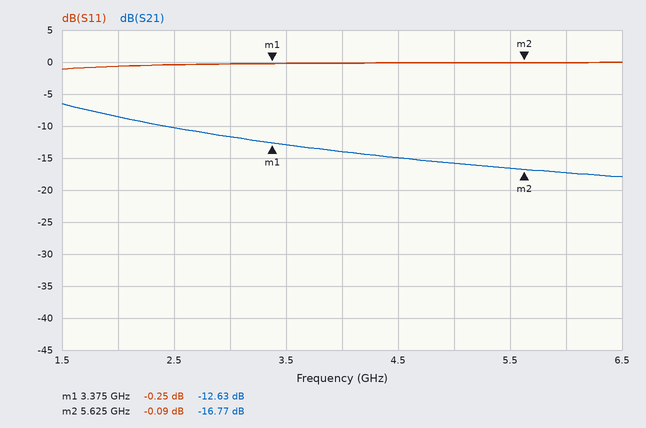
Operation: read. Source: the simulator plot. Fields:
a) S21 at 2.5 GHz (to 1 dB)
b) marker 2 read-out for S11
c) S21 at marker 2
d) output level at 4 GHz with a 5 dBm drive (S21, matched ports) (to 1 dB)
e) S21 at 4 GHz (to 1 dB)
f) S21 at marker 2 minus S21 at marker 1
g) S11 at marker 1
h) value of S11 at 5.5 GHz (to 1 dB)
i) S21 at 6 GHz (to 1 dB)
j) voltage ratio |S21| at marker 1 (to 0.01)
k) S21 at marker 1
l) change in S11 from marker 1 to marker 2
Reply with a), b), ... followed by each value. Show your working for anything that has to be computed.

a) -10 dB
b) -0.09 dB
c) -16.77 dB
d) 5 dBm + (-14 dB) = -9 dBm
e) -14 dB
f) -16.77 − (-12.63) = -4.14 dB
g) -0.25 dB
h) 0 dB
i) -17 dB
j) 10^(-12.63/20) ≈ 0.23
k) -12.63 dB
l) -0.09 − (-0.25) = 0.16 dB
